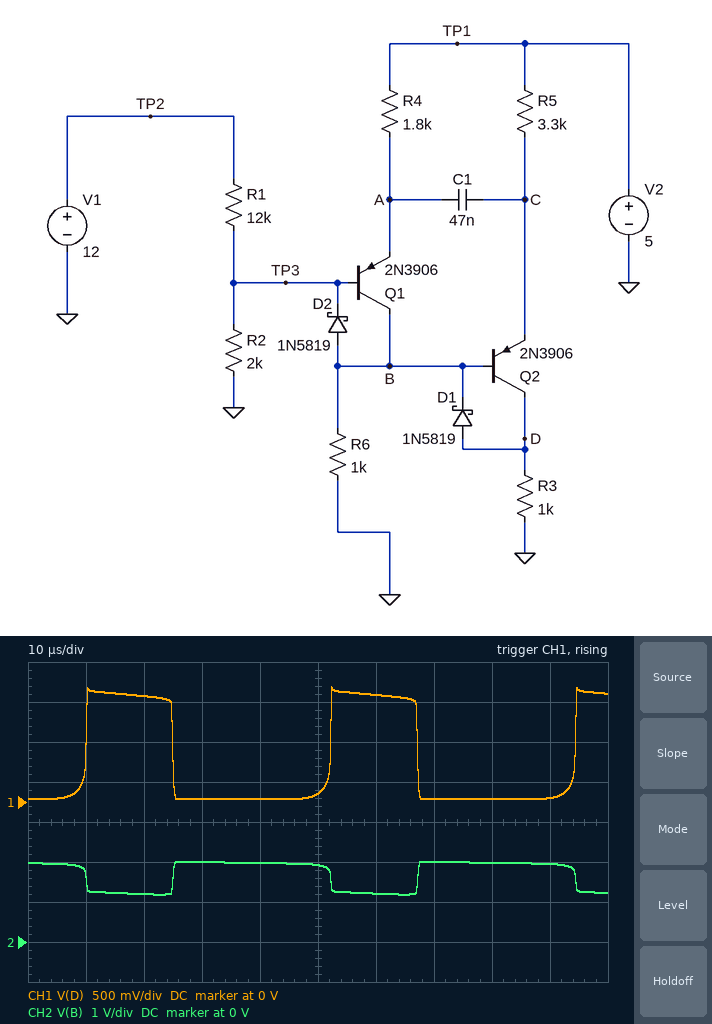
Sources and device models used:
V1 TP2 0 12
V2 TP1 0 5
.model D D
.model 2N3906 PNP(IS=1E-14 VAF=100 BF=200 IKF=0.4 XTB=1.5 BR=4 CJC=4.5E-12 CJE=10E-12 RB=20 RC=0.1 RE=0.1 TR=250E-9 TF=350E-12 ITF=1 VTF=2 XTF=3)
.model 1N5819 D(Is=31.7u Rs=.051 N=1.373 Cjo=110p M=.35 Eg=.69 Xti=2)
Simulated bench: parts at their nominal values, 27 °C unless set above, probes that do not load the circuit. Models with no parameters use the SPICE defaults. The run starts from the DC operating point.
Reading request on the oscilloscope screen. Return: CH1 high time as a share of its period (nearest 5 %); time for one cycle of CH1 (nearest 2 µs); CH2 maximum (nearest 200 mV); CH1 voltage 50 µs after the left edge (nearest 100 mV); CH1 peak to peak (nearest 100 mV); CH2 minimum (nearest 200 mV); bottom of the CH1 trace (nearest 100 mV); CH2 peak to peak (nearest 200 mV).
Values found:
35 %
42 µs
2.0 V
100 mV
1.4 V
1.2 V
0 V
800 mV
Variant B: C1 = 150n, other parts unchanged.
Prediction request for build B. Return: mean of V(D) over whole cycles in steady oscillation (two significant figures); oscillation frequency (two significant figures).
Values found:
500 mV
7.6 kHz
